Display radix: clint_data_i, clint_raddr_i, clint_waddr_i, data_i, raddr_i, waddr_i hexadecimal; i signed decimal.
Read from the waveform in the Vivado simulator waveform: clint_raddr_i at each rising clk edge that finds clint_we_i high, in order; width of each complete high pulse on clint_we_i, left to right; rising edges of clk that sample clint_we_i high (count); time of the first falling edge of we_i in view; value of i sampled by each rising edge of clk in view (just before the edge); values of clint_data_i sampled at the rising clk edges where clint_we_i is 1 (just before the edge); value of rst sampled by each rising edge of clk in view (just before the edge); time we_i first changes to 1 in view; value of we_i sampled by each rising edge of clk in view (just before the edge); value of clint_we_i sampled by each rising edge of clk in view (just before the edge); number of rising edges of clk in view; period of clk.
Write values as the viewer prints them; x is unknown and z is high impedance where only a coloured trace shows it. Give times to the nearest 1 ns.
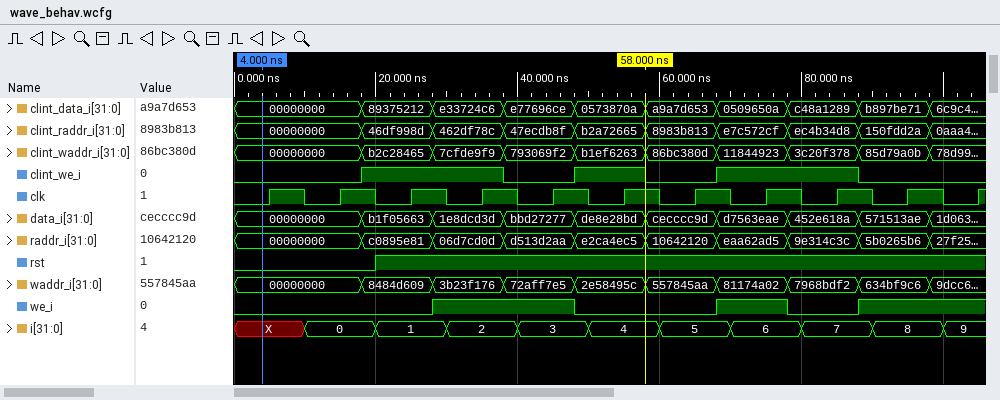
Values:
46df998d, 462df78c, b2a72665, e7c572cf, ec4b34d8
20 ns, 10 ns, 20 ns
5
48 ns
X, 0, 1, 2, 3, 4, 5, 6, 7, 8, 9
89375212, e33724c6, 0573870a, 0509650a, c48a1289
0 0 1 1 1 1 1 1 1 1 1
28 ns
0 0 0 1 1 0 0 1 0 1 1
0 0 1 1 0 1 0 1 1 0 0
11
10 ns
